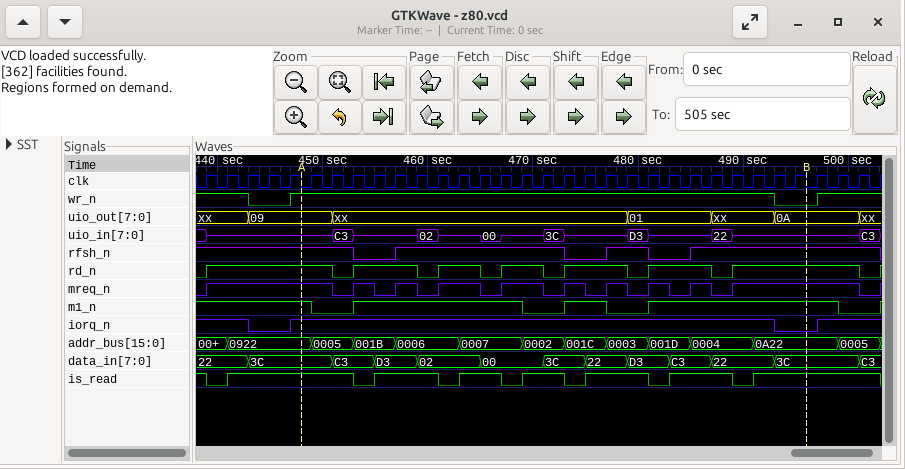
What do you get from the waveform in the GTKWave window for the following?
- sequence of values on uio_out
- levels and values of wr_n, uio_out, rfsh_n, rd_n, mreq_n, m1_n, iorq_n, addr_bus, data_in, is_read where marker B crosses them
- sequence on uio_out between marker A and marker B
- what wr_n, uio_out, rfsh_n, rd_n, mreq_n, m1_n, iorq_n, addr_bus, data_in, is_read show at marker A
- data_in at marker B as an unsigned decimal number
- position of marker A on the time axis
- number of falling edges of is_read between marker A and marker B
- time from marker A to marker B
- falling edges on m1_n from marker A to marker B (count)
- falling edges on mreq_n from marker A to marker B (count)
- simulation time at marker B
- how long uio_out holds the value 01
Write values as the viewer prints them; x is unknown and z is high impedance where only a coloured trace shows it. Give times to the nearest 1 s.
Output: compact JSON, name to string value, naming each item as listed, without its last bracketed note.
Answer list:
{"sequence of values on uio_out": "xx, 09, xx, 01, xx, 0A, xx", "levels and values of wr_n, uio_out, rfsh_n, rd_n, mreq_n, m1_n, iorq_n, addr_bus, data_in, is_read where marker B crosses them": "wr_n=0, uio_out=0A, rfsh_n=1, rd_n=1, mreq_n=1, m1_n=1, iorq_n=0, addr_bus=0A22, data_in=3C, is_read=1", "sequence on uio_out between marker A and marker B": "09, xx, 01, xx, 0A", "what wr_n, uio_out, rfsh_n, rd_n, mreq_n, m1_n, iorq_n, addr_bus, data_in, is_read show at marker A": "wr_n=1, uio_out=09, rfsh_n=1, rd_n=1, mreq_n=1, m1_n=1, iorq_n=1, addr_bus=0922, data_in=3C, is_read=1", "data_in at marker B as an unsigned decimal number": "60", "position of marker A on the time axis": "448 s", "number of falling edges of is_read between marker A and marker B": "6", "time from marker A to marker B": "48 s", "falling edges on m1_n from marker A to marker B": "3", "falling edges on mreq_n from marker A to marker B": "9", "simulation time at marker B": "496 s", "how long uio_out holds the value 01": "8 s"}
